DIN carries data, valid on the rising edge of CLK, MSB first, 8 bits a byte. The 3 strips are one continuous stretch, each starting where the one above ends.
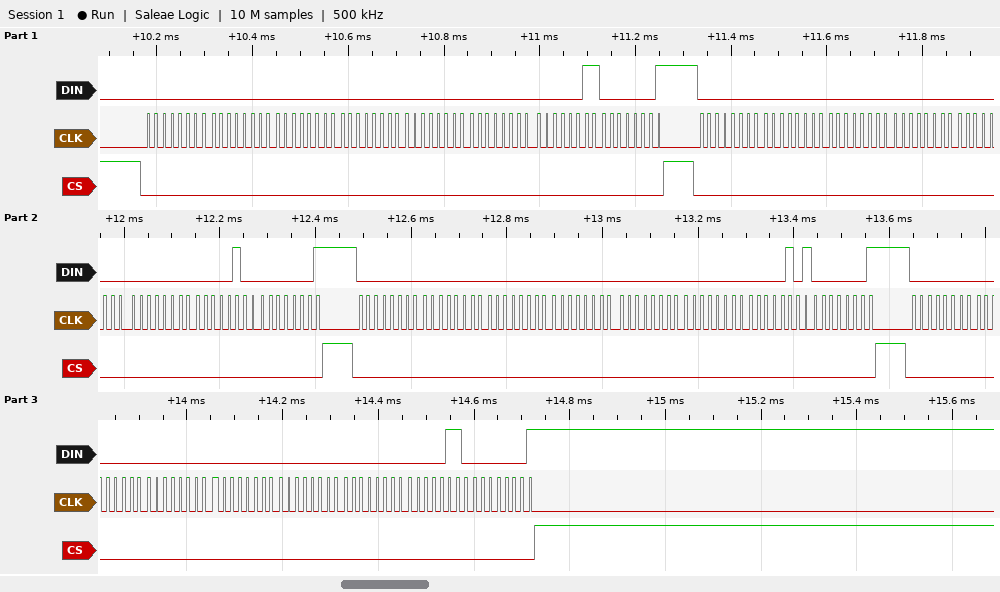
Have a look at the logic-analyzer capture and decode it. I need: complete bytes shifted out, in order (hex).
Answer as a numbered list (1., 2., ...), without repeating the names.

1. 00 00 00 00 00 00 03 01 00 00 00 00 00 00 04 01 00 00 00 00 00 00 05 01 00 00 00 00 00 00 06 01
